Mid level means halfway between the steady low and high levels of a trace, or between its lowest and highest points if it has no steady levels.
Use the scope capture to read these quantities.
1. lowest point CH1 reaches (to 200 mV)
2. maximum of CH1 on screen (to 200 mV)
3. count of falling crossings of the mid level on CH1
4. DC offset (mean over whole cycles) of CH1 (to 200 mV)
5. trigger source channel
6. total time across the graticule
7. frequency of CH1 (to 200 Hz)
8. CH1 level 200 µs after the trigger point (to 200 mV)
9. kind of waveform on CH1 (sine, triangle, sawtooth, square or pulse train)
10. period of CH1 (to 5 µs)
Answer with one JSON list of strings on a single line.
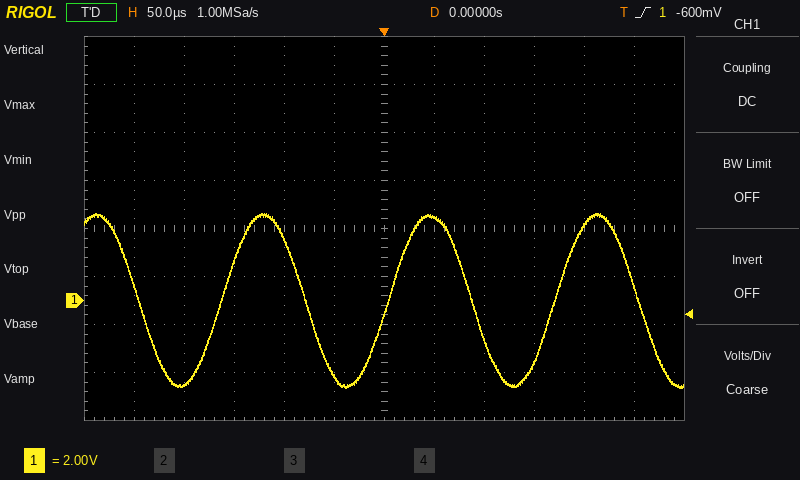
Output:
["-3.6 V", "3.6 V", "4", "0.0 V", "CH1", "600 µs", "6.0 kHz", "3.2 V", "sine", "165 µs"]
